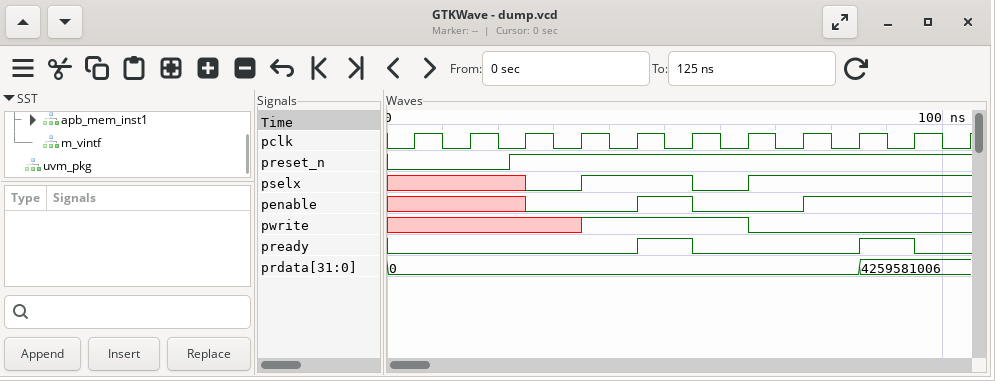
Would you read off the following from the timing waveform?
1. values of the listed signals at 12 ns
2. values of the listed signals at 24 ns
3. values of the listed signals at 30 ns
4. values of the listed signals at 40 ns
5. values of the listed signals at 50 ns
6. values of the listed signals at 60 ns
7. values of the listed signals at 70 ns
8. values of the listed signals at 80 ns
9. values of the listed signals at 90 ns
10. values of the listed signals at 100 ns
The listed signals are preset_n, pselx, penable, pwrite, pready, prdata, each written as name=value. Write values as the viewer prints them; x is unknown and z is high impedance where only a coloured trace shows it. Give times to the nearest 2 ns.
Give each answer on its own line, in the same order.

preset_n=0, pselx=x, penable=x, pwrite=x, pready=0, prdata=0
preset_n=1, pselx=x, penable=x, pwrite=x, pready=0, prdata=0
preset_n=1, pselx=0, penable=0, pwrite=x, pready=0, prdata=0
preset_n=1, pselx=1, penable=0, pwrite=1, pready=0, prdata=0
preset_n=1, pselx=1, penable=1, pwrite=1, pready=1, prdata=0
preset_n=1, pselx=0, penable=0, pwrite=1, pready=0, prdata=0
preset_n=1, pselx=1, penable=0, pwrite=0, pready=0, prdata=0
preset_n=1, pselx=1, penable=1, pwrite=0, pready=0, prdata=0
preset_n=1, pselx=1, penable=1, pwrite=0, pready=1, prdata=4259581006
preset_n=1, pselx=1, penable=1, pwrite=0, pready=0, prdata=4259581006
